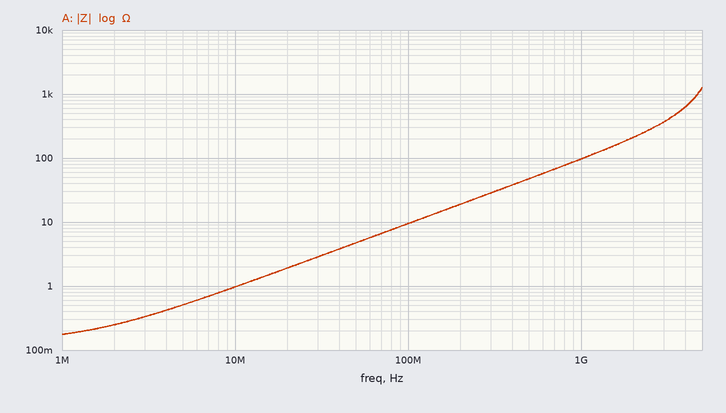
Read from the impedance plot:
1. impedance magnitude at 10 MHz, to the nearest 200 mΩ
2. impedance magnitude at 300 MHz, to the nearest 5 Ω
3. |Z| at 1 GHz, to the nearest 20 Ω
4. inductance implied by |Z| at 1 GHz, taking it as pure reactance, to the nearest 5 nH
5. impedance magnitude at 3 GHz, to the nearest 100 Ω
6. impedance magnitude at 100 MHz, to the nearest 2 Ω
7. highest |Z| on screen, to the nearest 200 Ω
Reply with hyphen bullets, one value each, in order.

- 1.0 Ω
- 30 Ω
- 100 Ω
- 15 nH
- 400 Ω
- 10 Ω
- 1.2 kΩ
